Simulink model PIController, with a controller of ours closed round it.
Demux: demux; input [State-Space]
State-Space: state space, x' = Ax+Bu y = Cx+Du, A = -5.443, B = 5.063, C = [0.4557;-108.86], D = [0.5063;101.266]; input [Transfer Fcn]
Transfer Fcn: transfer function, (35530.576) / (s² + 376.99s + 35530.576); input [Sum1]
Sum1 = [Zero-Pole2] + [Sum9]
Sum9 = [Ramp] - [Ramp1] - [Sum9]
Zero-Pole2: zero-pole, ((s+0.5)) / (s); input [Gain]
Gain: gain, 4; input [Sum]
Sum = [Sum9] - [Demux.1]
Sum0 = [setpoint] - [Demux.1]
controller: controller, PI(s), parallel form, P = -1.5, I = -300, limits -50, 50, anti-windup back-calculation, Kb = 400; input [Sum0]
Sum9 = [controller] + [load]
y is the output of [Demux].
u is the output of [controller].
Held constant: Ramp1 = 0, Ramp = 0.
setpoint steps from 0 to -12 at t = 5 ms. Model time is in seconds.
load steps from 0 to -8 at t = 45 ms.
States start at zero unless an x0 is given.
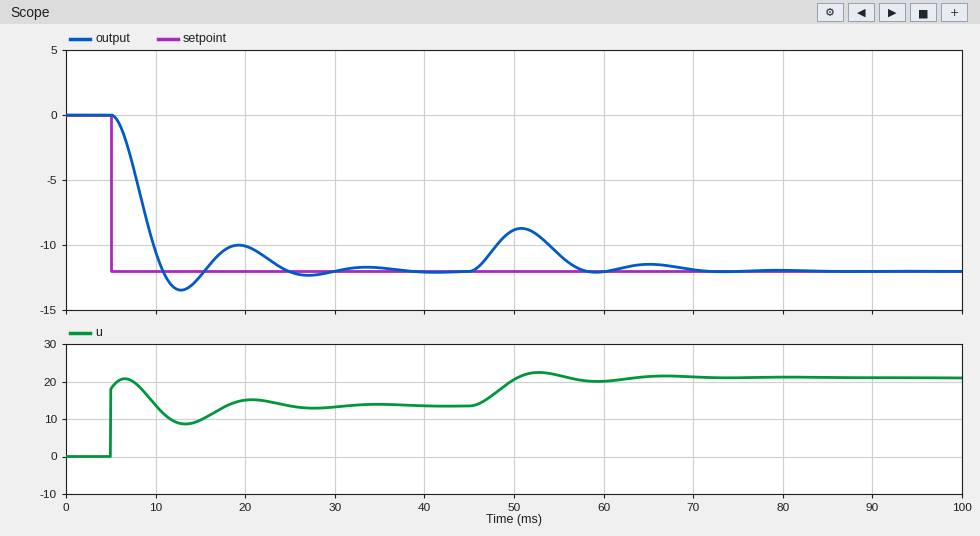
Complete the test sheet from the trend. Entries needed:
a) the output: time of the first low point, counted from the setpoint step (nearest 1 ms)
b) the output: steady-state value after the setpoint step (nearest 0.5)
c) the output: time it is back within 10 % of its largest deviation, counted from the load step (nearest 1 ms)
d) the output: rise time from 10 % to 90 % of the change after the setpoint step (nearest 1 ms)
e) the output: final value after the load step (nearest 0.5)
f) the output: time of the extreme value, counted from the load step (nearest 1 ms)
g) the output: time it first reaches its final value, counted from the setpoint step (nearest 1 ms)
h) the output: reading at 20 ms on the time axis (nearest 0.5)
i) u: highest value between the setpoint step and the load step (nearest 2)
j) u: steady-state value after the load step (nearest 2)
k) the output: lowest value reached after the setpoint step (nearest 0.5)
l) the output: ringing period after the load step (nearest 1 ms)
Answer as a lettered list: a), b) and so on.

a) 8 ms
b) -12.0
c) 23 ms
d) 4 ms
e) -12.0
f) 6 ms
g) 6 ms
h) -10.0
i) 20
j) 20
k) -13.5
l) 14 ms
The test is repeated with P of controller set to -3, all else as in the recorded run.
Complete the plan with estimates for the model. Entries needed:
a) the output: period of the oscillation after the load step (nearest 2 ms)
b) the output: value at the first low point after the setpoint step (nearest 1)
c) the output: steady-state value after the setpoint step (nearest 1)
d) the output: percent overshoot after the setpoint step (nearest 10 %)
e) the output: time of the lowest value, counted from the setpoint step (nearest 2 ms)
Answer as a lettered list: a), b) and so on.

a) 10 ms
b) -14
c) -12
d) 20 %
e) 6 ms
